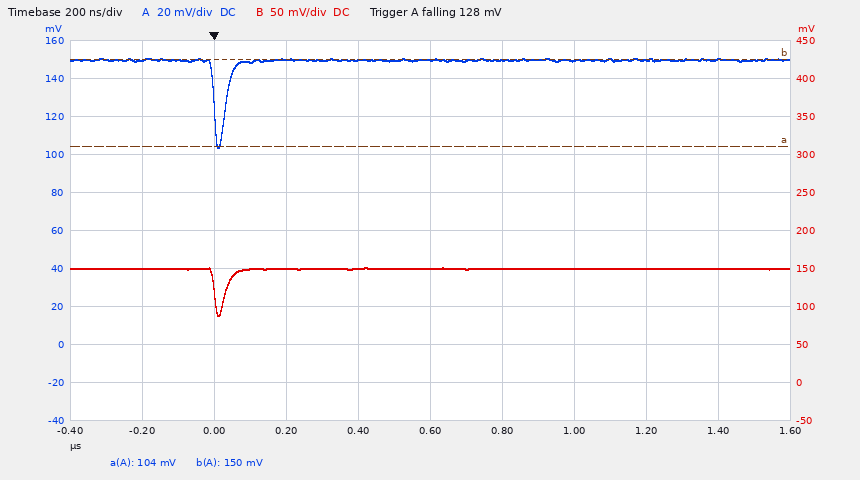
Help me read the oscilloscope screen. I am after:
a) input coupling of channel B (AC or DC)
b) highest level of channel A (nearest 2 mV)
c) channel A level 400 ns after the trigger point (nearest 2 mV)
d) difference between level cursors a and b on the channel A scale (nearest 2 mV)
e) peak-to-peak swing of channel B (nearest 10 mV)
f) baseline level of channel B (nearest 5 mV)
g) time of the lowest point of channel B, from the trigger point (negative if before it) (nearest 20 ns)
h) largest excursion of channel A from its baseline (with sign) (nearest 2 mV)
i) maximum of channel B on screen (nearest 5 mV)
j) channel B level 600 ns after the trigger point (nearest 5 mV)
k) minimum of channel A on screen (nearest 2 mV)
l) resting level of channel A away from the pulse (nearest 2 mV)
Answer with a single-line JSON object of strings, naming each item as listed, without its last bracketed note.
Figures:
{"input coupling of channel B": "DC", "highest level of channel A": "150 mV", "channel A level 400 ns after the trigger point": "150 mV", "difference between level cursors a and b on the channel A scale": "46 mV", "peak-to-peak swing of channel B": "60 mV", "baseline level of channel B": "150 mV", "time of the lowest point of channel B, from the trigger point (negative if before it)": "+20 ns", "largest excursion of channel A from its baseline (with sign)": "-46 mV", "maximum of channel B on screen": "150 mV", "channel B level 600 ns after the trigger point": "150 mV", "minimum of channel A on screen": "104 mV", "resting level of channel A away from the pulse": "150 mV"}
